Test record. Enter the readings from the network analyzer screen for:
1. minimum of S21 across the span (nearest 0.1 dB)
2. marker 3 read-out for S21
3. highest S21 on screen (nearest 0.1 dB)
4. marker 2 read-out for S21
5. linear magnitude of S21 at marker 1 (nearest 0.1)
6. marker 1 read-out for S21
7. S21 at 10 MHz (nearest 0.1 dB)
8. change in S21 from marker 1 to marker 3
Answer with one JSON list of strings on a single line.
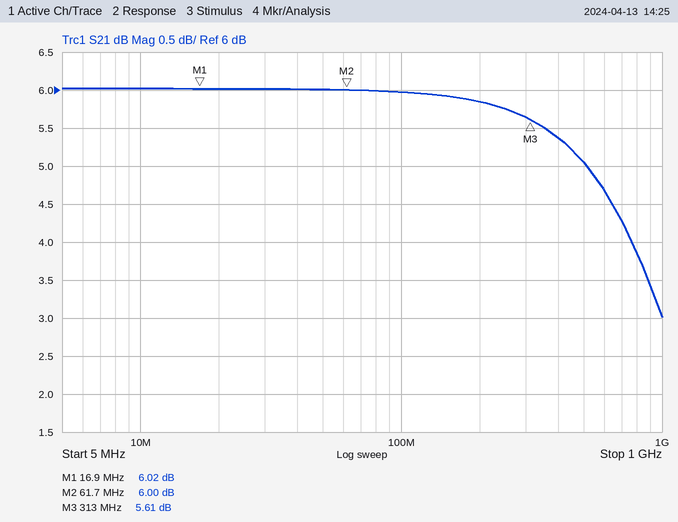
["3.0 dB", "5.61 dB", "6.0 dB", "6.00 dB", "2.0", "6.02 dB", "6.0 dB", "-0.41 dB"]
